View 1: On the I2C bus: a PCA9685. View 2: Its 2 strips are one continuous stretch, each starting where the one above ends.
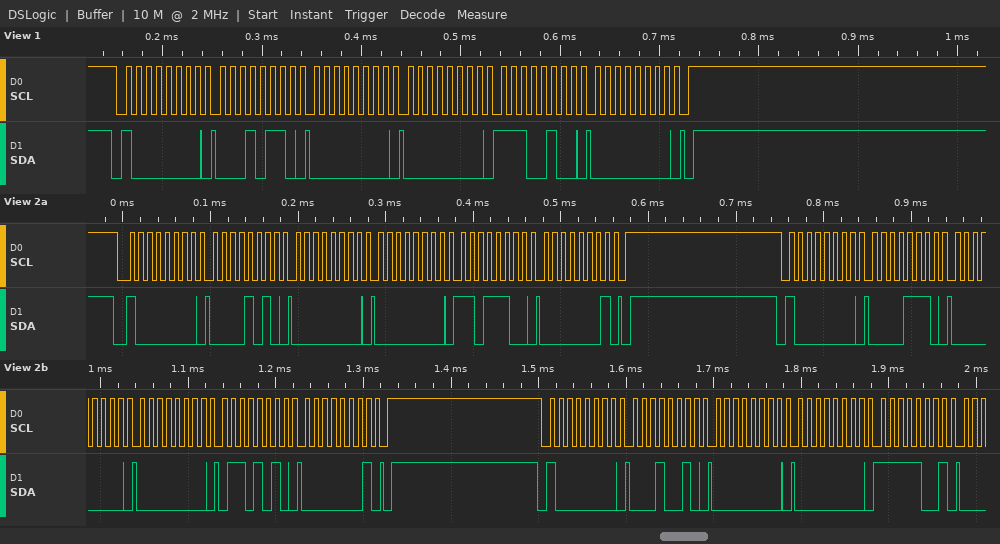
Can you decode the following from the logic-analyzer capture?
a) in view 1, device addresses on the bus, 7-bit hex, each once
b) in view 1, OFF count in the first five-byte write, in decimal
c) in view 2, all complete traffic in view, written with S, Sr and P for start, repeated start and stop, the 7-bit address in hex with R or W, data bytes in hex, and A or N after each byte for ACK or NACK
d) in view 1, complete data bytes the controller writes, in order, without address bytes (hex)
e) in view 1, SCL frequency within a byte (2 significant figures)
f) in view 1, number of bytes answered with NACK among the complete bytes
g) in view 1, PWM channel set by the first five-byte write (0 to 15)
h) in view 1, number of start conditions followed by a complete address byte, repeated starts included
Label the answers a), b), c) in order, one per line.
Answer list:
a) 0x40
b) 228
c) S 40W A 0A A 00 A 00 A DC A 01 A P S 40W A 0E A 00 A 00 A 6A A 01 A P S 40W A 12 A 00 A 00 A F9 A
d) 16 00 00 E4 00
e) 100 kHz
f) 0
g) 4
h) 1
